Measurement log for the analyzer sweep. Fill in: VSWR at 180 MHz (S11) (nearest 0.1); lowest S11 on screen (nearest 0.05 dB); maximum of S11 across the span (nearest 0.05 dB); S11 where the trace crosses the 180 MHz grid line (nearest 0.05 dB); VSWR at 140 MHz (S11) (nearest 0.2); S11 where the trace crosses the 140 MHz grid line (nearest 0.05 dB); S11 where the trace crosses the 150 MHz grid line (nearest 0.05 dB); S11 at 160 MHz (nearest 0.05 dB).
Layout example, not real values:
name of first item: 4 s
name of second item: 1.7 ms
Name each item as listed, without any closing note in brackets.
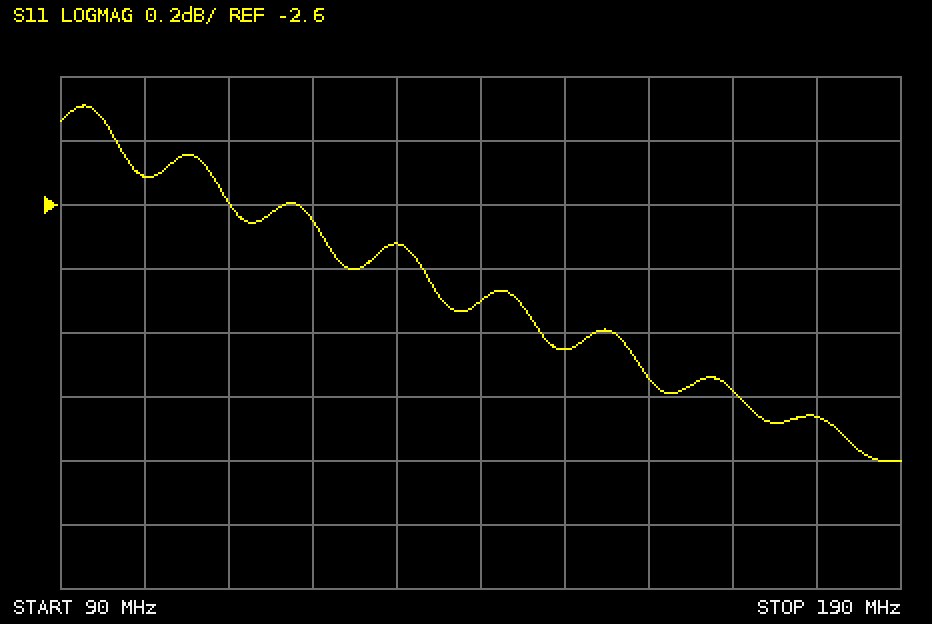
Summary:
VSWR at 180 MHz (S11): 5.4
lowest S11 on screen: -3.40 dB
maximum of S11 across the span: -2.30 dB
S11 where the trace crosses the 180 MHz grid line: -3.25 dB
VSWR at 140 MHz (S11): 6.0
S11 where the trace crosses the 140 MHz grid line: -2.90 dB
S11 where the trace crosses the 150 MHz grid line: -3.05 dB
S11 at 160 MHz: -3.15 dB
